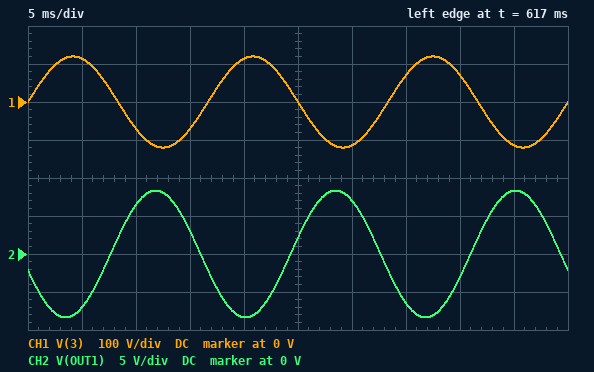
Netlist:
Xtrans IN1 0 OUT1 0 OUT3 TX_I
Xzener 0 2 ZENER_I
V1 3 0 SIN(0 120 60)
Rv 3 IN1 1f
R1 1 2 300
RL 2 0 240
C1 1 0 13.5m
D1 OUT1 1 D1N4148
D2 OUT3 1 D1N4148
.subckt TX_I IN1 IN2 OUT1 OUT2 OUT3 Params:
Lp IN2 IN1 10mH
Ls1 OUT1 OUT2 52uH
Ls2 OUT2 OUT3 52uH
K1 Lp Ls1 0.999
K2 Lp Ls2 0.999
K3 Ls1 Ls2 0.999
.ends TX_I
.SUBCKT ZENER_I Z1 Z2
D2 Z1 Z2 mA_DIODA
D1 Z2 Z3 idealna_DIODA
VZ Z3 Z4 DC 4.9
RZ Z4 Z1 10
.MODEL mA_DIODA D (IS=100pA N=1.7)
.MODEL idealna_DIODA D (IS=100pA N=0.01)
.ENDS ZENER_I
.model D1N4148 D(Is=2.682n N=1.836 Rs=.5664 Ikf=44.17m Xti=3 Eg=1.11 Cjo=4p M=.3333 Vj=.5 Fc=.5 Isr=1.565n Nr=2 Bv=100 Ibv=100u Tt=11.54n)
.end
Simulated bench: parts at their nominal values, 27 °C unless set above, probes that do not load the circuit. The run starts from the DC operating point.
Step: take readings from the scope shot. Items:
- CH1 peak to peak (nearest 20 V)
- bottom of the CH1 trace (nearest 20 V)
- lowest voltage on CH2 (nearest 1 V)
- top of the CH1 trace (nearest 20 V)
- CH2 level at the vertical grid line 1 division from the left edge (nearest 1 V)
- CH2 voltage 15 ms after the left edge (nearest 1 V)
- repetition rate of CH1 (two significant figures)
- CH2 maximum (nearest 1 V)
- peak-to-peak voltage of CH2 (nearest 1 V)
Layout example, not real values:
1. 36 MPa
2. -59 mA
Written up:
1. 240 V
2. -120 V
3. -8 V
4. 120 V
5. -7 V
6. 3 V
7. 60 Hz
8. 8 V
9. 17 V
